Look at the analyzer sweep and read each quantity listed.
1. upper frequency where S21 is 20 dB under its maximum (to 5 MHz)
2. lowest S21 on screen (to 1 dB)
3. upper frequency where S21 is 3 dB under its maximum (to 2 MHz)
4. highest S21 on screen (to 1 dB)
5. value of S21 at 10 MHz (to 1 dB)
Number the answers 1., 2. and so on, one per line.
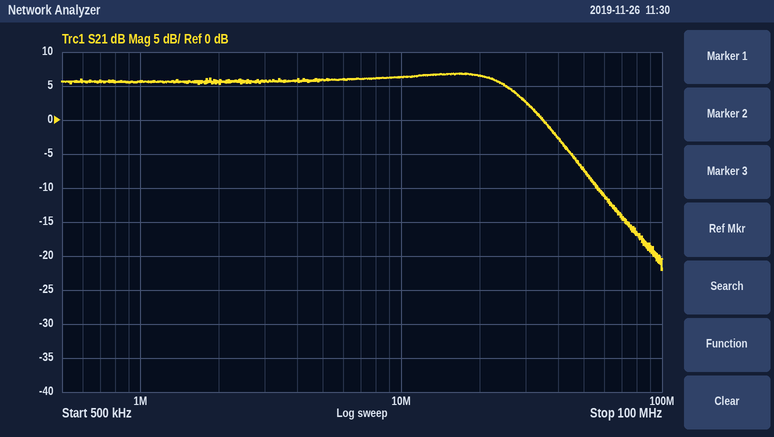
1. 65 MHz
2. -22 dB
3. 28 MHz
4. 7 dB
5. 6 dB
